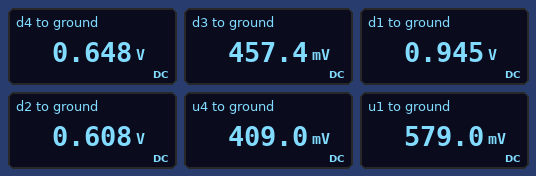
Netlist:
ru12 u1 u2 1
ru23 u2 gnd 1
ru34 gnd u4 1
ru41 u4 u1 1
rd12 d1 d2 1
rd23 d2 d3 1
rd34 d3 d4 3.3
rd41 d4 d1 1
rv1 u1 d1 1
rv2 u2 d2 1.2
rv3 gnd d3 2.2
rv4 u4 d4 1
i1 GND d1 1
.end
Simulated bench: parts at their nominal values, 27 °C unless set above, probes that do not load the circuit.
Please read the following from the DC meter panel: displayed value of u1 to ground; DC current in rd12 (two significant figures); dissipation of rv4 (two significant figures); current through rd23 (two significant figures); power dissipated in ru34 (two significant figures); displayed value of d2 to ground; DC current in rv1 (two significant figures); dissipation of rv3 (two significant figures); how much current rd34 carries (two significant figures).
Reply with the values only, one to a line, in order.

579.0 mV
340 mA
57 mW
150 mA
170 mW
0.608 V
370 mA
95 mW
58 mA
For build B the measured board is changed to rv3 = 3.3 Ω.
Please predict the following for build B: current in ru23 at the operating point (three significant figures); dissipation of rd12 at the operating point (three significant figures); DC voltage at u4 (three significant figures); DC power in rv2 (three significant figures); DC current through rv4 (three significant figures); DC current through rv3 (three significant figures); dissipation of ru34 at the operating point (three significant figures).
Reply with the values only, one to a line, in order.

407 mA
106 mW
430 mV
51.7 mW
254 mA
163 mA
185 mW
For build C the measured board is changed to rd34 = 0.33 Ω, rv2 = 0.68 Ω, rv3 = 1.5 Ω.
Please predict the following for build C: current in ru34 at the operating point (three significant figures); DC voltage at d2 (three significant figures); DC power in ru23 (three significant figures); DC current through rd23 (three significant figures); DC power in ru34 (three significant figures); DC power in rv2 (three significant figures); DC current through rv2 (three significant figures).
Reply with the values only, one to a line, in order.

339 mA
527 mV
139 mW
94.5 mA
115 mW
34.8 mW
226 mA
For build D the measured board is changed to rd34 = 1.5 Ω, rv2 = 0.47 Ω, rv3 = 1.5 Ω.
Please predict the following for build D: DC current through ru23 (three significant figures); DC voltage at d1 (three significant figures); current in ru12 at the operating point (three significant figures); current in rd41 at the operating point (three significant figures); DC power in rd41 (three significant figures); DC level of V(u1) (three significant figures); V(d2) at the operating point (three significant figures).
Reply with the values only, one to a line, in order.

388 mA
864 mV
151 mA
310 mA
96.3 mW
539 mV
499 mV
